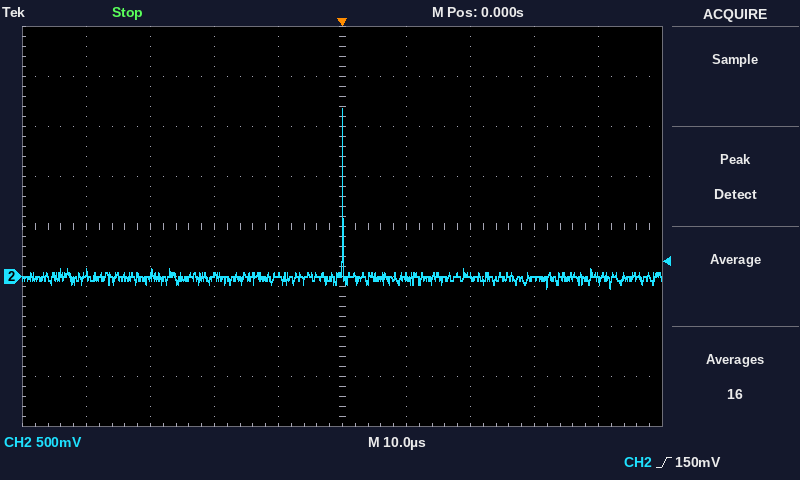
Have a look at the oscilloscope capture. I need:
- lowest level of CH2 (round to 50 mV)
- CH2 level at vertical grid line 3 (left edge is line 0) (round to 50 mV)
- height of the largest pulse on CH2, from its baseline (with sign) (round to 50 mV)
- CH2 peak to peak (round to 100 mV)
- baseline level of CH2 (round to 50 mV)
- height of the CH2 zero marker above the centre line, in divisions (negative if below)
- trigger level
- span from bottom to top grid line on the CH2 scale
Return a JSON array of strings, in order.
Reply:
["-100 mV", "0 mV", "+1.70 V", "1.80 V", "0 mV", "-1.0 div", "150 mV", "4 V"]
